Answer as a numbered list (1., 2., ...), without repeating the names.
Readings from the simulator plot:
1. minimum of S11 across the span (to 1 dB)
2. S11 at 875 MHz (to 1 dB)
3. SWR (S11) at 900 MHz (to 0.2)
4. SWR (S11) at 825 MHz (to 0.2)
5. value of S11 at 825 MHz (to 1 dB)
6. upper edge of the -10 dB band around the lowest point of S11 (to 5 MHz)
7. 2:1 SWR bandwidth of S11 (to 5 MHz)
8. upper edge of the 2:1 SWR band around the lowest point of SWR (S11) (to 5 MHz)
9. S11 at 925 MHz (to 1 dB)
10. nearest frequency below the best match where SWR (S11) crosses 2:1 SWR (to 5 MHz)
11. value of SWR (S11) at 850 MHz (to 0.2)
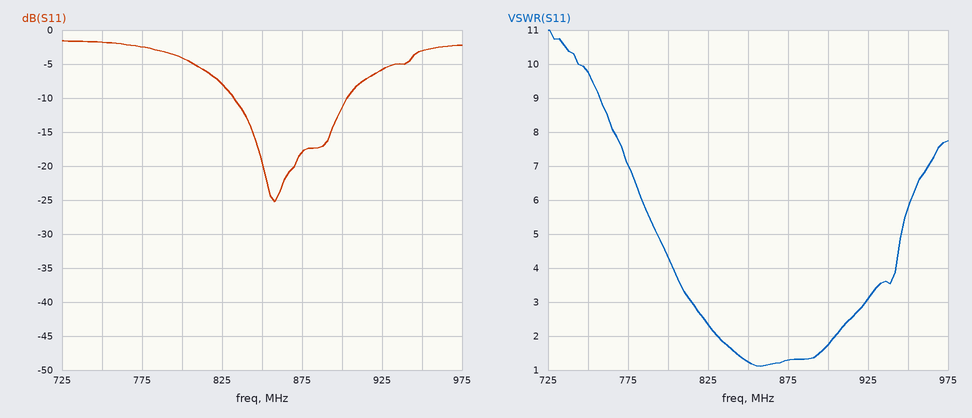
1. -25 dB
2. -18 dB
3. 1.8
4. 2.4
5. -8 dB
6. 905 MHz
7. 75 MHz
8. 905 MHz
9. -6 dB
10. 830 MHz
11. 1.2
